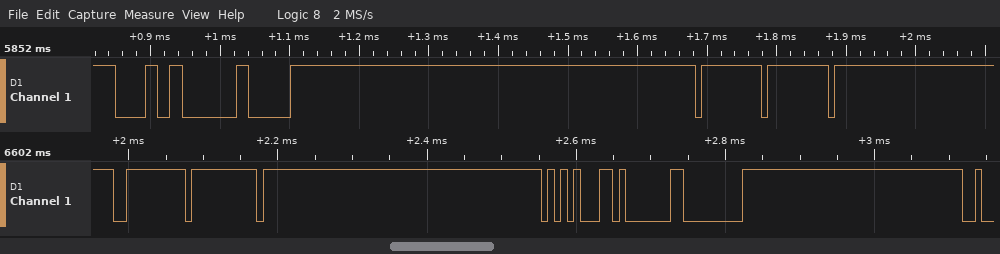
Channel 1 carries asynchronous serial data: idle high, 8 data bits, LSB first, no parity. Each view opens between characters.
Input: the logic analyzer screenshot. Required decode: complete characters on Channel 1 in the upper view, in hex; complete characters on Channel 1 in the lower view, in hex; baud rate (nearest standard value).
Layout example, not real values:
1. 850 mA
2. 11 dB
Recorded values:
1. 30, 00, C0, FF, FF, FF
2. FE, FF, FF, 15, 01, 00
3. 115200 baud
